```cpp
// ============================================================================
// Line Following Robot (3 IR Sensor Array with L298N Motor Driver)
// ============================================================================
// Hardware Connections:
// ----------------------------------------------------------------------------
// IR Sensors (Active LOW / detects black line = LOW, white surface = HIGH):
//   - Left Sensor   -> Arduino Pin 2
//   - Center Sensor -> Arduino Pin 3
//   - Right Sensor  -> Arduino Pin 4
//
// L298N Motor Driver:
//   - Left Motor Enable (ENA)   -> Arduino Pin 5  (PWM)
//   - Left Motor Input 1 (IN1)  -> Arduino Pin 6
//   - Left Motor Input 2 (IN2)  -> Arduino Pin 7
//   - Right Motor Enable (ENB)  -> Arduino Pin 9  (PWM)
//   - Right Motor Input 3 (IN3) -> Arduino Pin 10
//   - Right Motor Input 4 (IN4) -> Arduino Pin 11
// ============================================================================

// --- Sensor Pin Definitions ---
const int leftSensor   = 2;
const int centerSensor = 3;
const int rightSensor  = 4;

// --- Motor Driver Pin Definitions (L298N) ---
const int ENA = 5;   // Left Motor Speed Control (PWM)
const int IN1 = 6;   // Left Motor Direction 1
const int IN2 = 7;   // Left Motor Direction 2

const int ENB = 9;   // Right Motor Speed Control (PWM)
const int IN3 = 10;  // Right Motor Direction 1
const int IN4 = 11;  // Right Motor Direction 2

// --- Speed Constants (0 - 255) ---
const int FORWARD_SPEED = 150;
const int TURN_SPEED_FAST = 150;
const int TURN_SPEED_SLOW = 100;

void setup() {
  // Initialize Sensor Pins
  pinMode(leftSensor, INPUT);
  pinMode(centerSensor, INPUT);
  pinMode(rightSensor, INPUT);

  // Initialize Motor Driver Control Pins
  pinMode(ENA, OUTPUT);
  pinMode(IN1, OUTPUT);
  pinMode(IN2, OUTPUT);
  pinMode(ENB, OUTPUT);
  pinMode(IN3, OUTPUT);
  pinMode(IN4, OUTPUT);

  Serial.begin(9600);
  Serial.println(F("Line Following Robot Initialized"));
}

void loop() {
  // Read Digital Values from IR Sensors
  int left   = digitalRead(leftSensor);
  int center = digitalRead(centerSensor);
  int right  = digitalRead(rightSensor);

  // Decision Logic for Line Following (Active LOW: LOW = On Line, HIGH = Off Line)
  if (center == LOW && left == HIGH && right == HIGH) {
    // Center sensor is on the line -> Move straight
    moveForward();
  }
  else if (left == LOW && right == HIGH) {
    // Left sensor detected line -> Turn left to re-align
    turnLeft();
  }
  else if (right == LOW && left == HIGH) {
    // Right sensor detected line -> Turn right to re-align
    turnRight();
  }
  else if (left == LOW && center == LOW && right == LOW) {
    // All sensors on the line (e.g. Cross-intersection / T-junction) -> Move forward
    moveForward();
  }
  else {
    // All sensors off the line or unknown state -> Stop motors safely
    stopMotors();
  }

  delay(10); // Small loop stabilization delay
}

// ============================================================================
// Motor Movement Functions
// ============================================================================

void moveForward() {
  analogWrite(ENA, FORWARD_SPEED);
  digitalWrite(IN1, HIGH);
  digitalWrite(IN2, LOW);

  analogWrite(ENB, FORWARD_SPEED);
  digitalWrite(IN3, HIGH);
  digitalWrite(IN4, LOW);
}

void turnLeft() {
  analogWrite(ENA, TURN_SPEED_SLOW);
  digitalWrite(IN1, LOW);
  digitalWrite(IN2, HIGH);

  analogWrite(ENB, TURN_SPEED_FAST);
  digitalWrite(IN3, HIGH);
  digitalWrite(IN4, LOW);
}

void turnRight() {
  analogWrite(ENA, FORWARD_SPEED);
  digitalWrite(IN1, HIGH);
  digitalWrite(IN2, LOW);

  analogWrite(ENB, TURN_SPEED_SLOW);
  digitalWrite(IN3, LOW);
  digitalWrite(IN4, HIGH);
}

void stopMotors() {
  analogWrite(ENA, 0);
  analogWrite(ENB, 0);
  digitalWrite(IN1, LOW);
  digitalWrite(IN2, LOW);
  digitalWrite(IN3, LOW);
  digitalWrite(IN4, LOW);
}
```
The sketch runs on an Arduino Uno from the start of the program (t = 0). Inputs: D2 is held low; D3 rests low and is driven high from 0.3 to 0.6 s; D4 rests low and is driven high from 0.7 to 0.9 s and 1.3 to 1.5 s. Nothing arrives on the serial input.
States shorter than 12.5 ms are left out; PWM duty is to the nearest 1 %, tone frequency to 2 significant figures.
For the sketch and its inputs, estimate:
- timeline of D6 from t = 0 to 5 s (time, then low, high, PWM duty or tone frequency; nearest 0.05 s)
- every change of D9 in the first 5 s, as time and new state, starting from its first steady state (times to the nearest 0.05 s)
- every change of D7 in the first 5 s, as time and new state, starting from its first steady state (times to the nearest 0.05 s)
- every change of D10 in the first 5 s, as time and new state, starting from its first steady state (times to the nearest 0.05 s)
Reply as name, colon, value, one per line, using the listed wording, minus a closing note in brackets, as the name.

timeline of D6 from t = 0 to 5 s: 0 s high; 0.3 s low; 0.6 s high; 0.7 s low; 0.9 s high; 1.3 s low; 1.5 s high
every change of D9 in the first 5 s, as time and new state, starting from its first steady state: 0 s PWM 59 %; 0.3 s low; 0.6 s PWM 59 %
every change of D7 in the first 5 s, as time and new state, starting from its first steady state: 0 s low; 0.7 s high; 0.9 s low; 1.3 s high; 1.5 s low
every change of D10 in the first 5 s, as time and new state, starting from its first steady state: 0 s high; 0.3 s low; 0.6 s high
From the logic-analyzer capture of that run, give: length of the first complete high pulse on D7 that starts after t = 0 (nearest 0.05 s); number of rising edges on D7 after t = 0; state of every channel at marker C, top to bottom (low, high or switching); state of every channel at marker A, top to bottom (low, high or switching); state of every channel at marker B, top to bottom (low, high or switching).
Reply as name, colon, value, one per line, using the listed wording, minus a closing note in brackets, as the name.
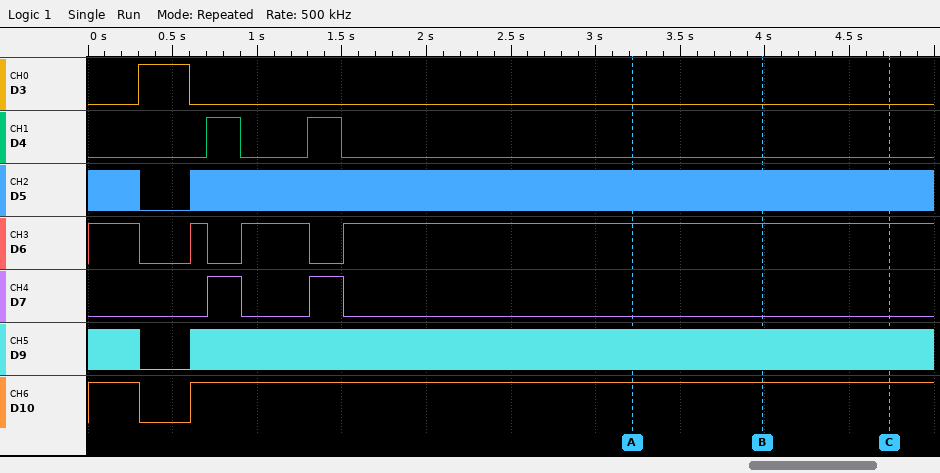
length of the first complete high pulse on D7 that starts after t = 0: 0.20 s
number of rising edges on D7 after t = 0: 2
state of every channel at marker C, top to bottom: D3 low, D4 low, D5 switching, D6 high, D7 low, D9 switching, D10 high
state of every channel at marker A, top to bottom: D3 low, D4 low, D5 switching, D6 high, D7 low, D9 switching, D10 high
state of every channel at marker B, top to bottom: D3 low, D4 low, D5 switching, D6 high, D7 low, D9 switching, D10 high
